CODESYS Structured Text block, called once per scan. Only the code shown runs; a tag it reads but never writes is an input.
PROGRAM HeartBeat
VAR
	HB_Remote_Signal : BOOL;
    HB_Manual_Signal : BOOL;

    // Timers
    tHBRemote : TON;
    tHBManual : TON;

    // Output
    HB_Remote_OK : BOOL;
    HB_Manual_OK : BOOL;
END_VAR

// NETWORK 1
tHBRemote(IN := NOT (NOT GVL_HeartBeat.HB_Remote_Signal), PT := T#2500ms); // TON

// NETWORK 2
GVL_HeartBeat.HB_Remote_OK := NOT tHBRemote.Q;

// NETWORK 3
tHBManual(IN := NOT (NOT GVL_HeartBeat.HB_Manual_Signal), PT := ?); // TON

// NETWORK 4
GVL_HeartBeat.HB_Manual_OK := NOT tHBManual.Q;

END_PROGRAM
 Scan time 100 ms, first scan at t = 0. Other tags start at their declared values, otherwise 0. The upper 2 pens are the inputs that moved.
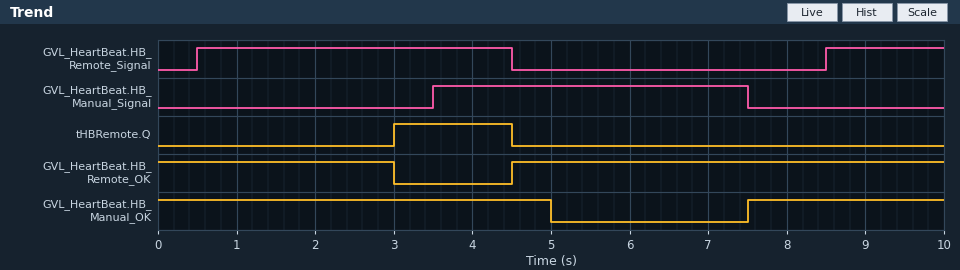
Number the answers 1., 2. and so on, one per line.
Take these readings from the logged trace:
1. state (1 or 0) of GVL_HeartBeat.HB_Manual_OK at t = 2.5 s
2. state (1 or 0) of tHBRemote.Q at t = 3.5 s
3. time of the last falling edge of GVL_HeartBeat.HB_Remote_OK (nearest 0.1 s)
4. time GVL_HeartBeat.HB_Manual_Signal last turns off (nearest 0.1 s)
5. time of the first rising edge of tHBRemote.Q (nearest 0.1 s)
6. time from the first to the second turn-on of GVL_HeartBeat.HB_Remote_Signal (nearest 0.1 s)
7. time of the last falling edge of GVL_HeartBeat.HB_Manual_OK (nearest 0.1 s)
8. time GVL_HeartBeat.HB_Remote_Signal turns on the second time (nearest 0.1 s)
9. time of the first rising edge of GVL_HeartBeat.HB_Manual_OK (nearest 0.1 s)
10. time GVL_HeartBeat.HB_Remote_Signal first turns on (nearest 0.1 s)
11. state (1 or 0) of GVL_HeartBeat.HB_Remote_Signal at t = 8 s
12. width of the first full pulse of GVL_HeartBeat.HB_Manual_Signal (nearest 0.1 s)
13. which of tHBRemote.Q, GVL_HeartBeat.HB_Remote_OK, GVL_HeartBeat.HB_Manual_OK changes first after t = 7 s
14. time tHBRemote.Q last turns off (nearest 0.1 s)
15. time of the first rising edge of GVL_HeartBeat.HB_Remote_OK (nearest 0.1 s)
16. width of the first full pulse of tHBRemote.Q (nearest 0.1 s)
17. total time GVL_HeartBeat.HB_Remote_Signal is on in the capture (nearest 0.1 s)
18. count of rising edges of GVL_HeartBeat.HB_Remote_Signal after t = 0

1. 1
2. 1
3. 3.0 s
4. 7.5 s
5. 3.0 s
6. 8.0 s
7. 5.0 s
8. 8.5 s
9. 7.5 s
10. 0.5 s
11. 0
12. 4.0 s
13. GVL_HeartBeat.HB_Manual_OK
14. 4.5 s
15. 4.5 s
16. 1.5 s
17. 5.5 s
18. 2
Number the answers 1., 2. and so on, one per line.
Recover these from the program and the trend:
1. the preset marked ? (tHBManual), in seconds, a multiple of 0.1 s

1. 1.5 s
